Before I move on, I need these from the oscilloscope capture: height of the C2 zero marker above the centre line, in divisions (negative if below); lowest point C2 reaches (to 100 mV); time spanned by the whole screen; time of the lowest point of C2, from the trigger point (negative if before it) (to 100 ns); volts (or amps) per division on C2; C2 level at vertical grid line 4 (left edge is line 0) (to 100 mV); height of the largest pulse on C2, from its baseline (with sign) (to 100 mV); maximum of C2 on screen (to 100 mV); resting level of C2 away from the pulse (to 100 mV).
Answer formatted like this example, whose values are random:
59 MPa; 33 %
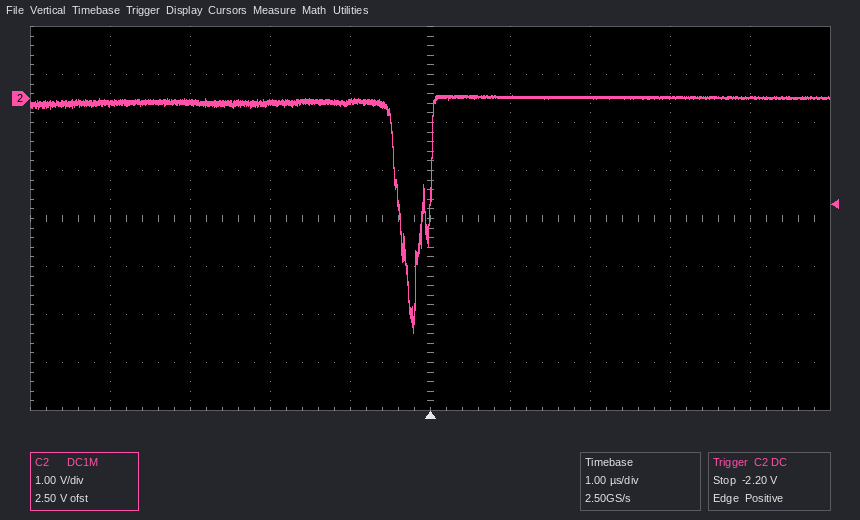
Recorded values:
+2.5 div; -4.9 V; 10 µs; -200 ns; 1 V; -100 mV; -4.9 V; 100 mV; 0.0 V
